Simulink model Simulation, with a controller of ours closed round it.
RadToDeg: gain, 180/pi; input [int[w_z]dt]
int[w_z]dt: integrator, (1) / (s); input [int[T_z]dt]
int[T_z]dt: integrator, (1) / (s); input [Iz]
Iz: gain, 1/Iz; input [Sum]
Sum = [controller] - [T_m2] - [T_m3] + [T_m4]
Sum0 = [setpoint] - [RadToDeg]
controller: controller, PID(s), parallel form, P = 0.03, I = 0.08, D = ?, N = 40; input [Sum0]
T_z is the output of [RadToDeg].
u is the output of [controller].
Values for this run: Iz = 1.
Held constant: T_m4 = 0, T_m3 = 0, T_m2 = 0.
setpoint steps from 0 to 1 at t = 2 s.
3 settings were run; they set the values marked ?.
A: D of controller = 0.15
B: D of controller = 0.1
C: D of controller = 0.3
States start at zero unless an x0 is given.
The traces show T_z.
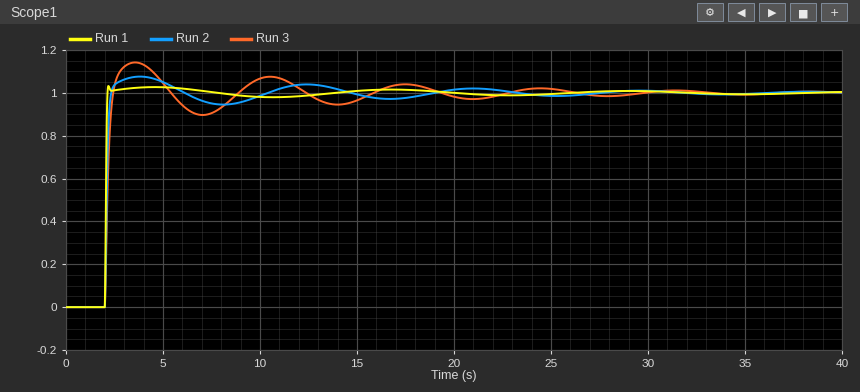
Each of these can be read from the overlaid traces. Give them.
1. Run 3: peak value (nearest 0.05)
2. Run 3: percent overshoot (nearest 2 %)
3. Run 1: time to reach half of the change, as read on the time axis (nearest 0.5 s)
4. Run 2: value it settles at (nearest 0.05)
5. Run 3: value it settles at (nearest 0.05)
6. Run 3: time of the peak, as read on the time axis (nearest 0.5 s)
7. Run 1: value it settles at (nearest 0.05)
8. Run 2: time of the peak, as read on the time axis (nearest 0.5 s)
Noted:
1.15
14 %
2.0 s
1.00
1.00
3.5 s
1.00
4.0 s
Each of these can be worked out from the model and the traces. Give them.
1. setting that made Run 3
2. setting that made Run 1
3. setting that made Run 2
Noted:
B
C
A
